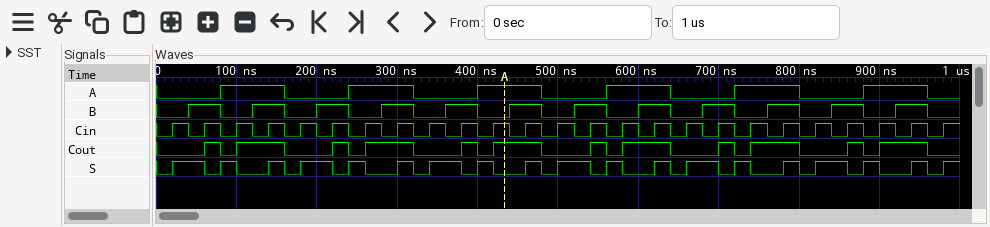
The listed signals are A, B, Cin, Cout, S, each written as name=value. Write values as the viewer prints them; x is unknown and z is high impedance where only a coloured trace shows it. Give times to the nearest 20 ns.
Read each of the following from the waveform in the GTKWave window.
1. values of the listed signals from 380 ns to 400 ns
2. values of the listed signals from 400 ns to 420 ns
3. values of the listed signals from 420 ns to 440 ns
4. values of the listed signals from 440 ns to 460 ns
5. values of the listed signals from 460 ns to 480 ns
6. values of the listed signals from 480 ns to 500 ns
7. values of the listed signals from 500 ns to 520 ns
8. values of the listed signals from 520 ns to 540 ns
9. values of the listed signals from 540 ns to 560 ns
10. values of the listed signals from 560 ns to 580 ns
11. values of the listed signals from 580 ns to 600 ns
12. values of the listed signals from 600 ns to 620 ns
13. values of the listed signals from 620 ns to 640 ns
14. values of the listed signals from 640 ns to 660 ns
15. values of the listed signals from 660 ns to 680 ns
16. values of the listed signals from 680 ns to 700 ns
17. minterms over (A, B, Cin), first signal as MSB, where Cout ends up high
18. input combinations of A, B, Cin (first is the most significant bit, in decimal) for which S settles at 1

A=0, B=1, Cin=1, Cout=1, S=0
A=1, B=0, Cin=0, Cout=0, S=1
A=1, B=0, Cin=1, Cout=1, S=0
A=1, B=1, Cin=0, Cout=1, S=0
A=1, B=1, Cin=1, Cout=1, S=1
A=0, B=0, Cin=0, Cout=0, S=0
A=0, B=0, Cin=1, Cout=0, S=1
A=0, B=1, Cin=0, Cout=0, S=1
A=0, B=1, Cin=1, Cout=1, S=0
A=1, B=0, Cin=0, Cout=0, S=1
A=1, B=0, Cin=1, Cout=1, S=0
A=1, B=1, Cin=0, Cout=1, S=0
A=1, B=1, Cin=1, Cout=1, S=1
A=0, B=0, Cin=0, Cout=0, S=0
A=0, B=0, Cin=1, Cout=0, S=1
A=0, B=1, Cin=0, Cout=0, S=1
3, 5, 6, 7
1, 2, 4, 7
